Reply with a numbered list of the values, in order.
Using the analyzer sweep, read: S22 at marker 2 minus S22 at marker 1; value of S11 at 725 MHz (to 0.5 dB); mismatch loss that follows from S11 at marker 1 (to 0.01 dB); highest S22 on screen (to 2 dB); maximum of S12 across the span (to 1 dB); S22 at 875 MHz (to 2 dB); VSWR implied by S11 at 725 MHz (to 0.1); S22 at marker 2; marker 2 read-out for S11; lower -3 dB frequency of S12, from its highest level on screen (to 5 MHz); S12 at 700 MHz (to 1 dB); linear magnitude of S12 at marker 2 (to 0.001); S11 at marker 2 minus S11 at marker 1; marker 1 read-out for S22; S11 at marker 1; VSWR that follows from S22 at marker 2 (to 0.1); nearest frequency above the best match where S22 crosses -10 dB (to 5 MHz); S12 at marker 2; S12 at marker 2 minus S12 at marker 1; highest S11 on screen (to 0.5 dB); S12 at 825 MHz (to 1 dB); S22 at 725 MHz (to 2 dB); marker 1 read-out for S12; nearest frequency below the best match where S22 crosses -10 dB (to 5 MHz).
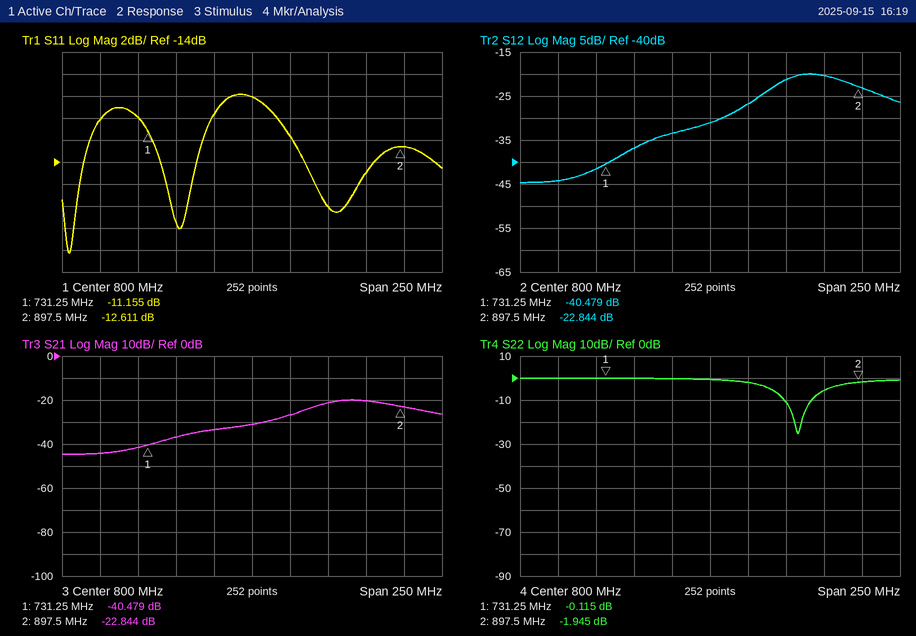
1. -1.830 dB
2. -10.0 dB
3. 0.35 dB
4. 0 dB
5. -20 dB
6. -6 dB
7. 1.9
8. -1.945 dB
9. -12.611 dB
10. 840 MHz
11. -44 dB
12. 0.072
13. -1.456 dB
14. -0.115 dB
15. -11.155 dB
16. 9.0
17. 865 MHz
18. -22.844 dB
19. 17.635 dB
20. -8.0 dB
21. -27 dB
22. 0 dB
23. -40.479 dB
24. 850 MHz
